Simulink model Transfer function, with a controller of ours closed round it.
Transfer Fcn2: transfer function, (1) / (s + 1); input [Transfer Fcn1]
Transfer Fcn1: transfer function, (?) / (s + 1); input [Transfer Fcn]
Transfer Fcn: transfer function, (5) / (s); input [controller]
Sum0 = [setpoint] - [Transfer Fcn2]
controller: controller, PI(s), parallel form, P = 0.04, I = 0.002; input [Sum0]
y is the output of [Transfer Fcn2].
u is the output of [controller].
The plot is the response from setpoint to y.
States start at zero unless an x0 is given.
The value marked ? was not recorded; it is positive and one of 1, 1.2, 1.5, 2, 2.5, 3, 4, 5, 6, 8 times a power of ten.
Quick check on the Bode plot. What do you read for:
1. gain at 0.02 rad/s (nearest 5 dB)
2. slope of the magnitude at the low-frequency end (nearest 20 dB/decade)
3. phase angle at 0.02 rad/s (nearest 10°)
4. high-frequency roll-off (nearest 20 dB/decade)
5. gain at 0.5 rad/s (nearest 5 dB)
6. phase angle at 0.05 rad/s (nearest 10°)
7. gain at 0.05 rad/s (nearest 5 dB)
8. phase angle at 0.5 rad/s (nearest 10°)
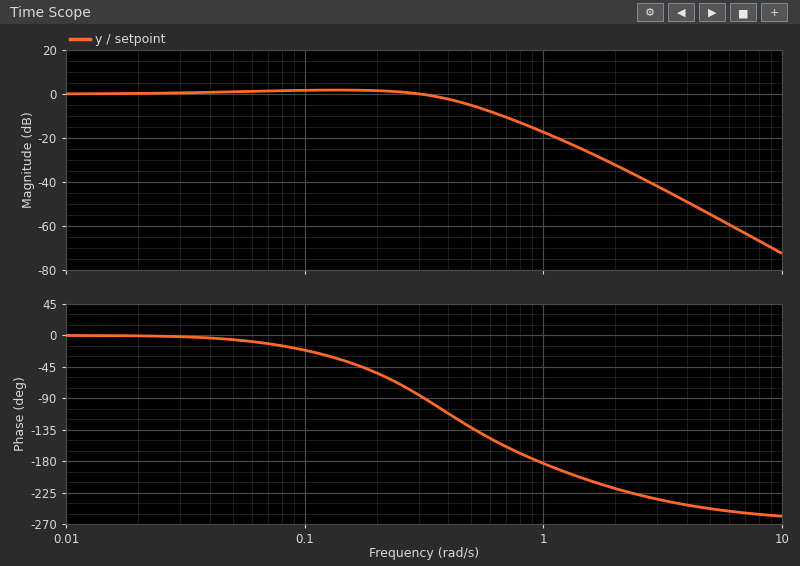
0 dB
0 dB/decade
0°
-60 dB/decade
-5 dB
-10°
0 dB
-130°
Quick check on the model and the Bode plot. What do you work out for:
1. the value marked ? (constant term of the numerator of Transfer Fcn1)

1.2
